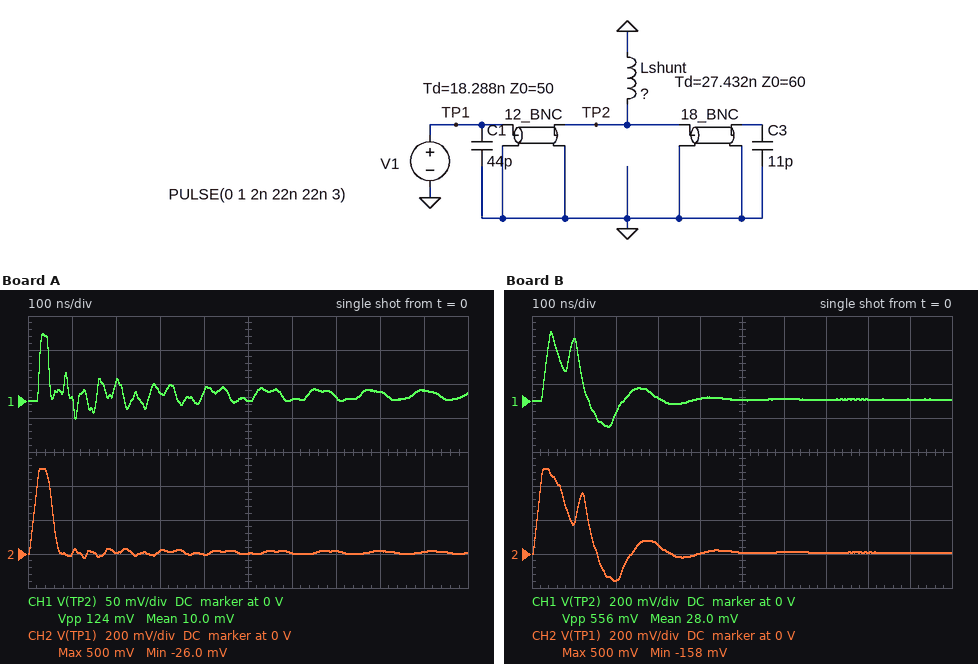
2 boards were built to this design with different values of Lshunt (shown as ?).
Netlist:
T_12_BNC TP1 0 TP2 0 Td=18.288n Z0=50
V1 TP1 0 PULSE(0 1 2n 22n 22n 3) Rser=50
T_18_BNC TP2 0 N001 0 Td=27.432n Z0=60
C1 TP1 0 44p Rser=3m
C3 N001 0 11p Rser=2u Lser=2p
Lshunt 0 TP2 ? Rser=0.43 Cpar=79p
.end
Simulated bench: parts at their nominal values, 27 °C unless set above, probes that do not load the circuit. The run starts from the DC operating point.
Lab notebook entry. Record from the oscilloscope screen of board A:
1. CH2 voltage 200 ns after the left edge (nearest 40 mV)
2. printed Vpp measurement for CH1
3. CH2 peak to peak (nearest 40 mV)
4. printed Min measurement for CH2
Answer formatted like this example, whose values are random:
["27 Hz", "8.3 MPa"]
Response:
["0 V", "124 mV", "520 mV", "-26.0 mV"]
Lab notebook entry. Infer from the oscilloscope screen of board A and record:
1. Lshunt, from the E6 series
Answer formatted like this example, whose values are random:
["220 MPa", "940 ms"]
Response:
["100 nH"]
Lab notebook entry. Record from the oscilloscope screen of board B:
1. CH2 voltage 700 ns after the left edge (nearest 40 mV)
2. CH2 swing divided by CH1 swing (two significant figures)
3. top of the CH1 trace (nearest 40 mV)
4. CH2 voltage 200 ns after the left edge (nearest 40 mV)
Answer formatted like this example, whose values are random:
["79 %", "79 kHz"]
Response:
["0 V", "1.2", "400 mV", "-160 mV"]
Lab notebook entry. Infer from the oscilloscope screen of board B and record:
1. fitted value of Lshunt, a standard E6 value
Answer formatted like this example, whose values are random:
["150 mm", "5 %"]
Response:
["1 µH"]
